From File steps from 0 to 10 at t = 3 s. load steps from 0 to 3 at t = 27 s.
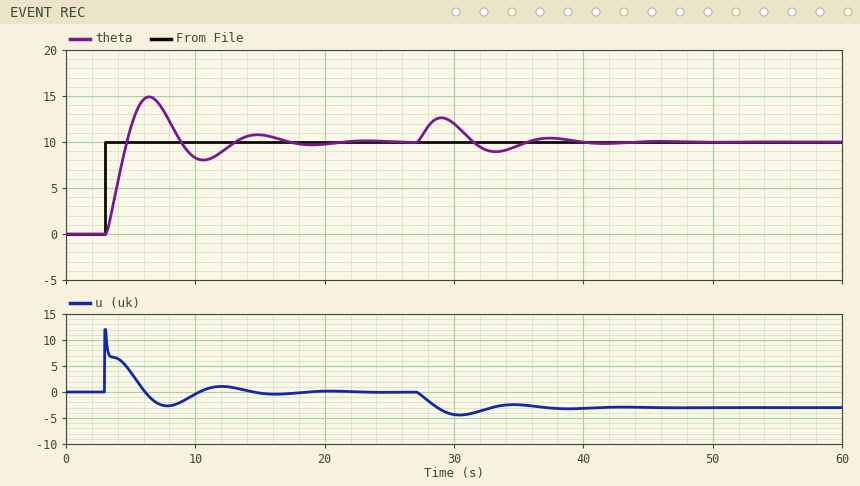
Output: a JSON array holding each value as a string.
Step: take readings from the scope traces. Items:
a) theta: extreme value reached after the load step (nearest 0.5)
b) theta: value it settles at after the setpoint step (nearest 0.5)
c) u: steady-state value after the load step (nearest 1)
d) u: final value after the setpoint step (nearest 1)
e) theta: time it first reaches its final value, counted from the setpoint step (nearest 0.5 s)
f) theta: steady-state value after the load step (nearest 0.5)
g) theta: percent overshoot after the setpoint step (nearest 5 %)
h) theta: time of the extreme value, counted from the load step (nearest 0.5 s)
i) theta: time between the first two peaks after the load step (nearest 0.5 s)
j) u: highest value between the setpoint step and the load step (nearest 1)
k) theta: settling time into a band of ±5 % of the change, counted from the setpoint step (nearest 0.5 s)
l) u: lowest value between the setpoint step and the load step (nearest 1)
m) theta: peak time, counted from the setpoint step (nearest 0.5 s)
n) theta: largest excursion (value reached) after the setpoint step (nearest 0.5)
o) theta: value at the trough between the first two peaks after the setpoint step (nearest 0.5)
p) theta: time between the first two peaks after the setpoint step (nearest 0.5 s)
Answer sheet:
["12.5", "10.0", "-3", "0", "1.5 s", "10.0", "50 %", "2.0 s", "8.5 s", "12", "13.0 s", "-3", "3.5 s", "15.0", "8.0", "8.5 s"]
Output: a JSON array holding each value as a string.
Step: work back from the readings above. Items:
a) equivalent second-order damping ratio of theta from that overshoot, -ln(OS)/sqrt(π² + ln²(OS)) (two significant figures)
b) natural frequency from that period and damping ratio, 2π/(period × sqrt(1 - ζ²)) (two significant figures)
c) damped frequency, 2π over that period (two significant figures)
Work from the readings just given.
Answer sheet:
["0.22", "0.76 rad/s", "0.74 rad/s"]
